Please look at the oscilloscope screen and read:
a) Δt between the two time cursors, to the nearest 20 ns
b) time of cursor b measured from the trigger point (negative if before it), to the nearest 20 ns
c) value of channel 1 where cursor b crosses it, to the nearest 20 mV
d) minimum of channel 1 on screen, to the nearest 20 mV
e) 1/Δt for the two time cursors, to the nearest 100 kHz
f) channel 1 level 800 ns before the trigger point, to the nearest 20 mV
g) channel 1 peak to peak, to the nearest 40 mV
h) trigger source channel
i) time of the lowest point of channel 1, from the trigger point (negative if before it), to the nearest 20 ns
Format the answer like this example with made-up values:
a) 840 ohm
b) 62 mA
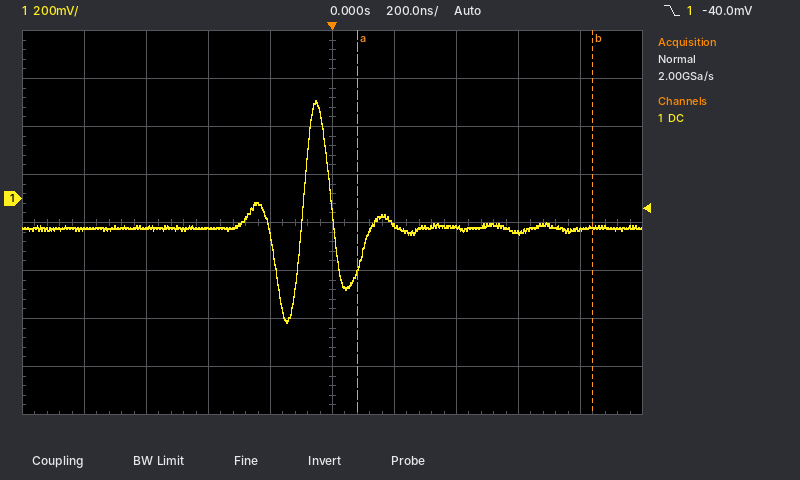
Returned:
a) 760 ns
b) +840 ns
c) -120 mV
d) -520 mV
e) 1.3 MHz
f) -120 mV
g) 920 mV
h) channel 1
i) -140 ns
